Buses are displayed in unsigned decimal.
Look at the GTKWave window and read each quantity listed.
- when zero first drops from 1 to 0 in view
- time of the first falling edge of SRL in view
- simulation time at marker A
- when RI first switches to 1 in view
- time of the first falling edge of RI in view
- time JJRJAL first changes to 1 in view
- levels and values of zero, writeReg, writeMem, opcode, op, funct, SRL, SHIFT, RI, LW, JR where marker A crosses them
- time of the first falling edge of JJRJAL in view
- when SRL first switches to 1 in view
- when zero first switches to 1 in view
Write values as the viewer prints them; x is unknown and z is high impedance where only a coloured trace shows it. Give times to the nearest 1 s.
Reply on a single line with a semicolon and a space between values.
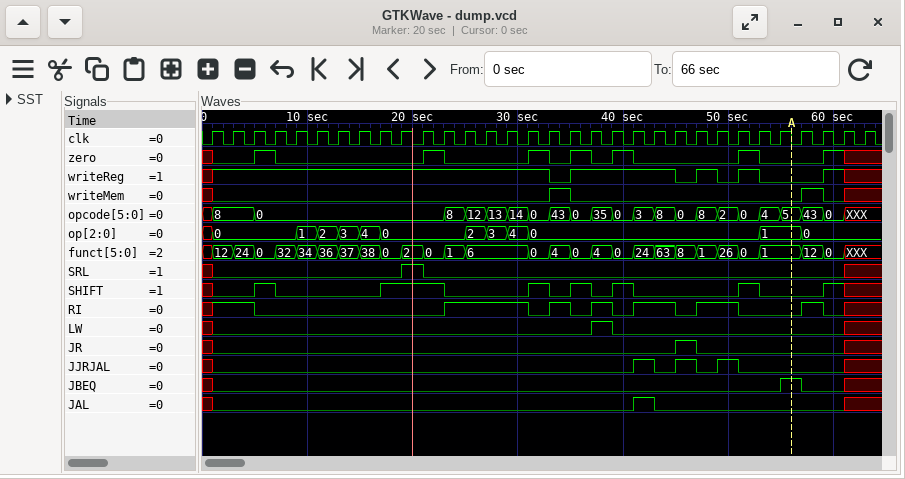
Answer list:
7 s; 21 s; 56 s; 1 s; 5 s; 41 s; zero=0, writeReg=0, writeMem=0, opcode=5, op=1, funct=1, SRL=0, SHIFT=0, RI=0, LW=0, JR=0; 43 s; 19 s; 5 s
